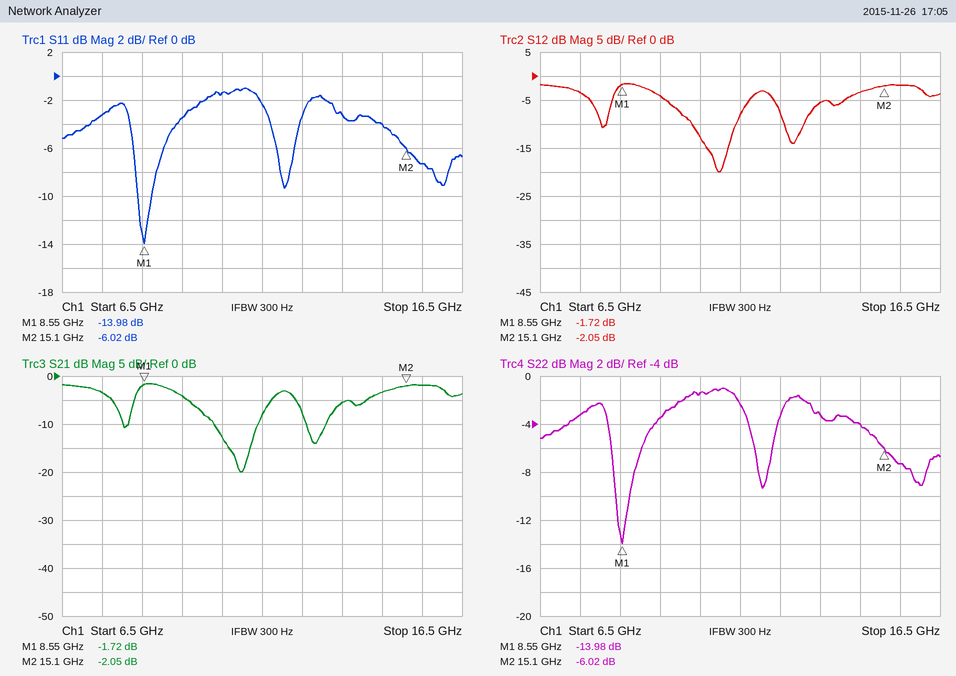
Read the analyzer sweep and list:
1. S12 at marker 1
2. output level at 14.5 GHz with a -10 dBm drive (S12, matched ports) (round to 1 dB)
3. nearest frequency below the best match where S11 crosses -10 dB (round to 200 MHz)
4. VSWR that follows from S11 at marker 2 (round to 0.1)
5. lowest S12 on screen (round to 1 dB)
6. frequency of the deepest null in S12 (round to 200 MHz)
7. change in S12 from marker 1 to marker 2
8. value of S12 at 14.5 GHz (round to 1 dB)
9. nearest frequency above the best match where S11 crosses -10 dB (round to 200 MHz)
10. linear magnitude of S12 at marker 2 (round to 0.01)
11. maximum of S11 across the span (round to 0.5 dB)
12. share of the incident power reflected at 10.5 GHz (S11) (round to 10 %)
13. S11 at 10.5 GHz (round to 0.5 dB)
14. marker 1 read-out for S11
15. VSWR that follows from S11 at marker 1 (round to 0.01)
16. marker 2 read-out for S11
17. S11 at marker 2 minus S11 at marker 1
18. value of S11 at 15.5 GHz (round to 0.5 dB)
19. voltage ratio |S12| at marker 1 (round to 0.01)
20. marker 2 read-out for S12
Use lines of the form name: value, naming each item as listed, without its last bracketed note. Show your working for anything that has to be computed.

S12 at marker 1: -1.72 dB
output level at 14.5 GHz with a -10 dBm drive (S12, matched ports): -10 dBm + (-3 dB) = -13 dBm
nearest frequency below the best match where S11 crosses -10 dB: 8.4 GHz
VSWR that follows from S11 at marker 2: (1 + 0.5000)/(1 − 0.5000) ≈ 3.0
lowest S12 on screen: -20 dB
frequency of the deepest null in S12: 11.0 GHz
change in S12 from marker 1 to marker 2: -2.05 − (-1.72) = -0.33 dB
value of S12 at 14.5 GHz: -3 dB
nearest frequency above the best match where S11 crosses -10 dB: 8.8 GHz
linear magnitude of S12 at marker 2: 10^(-2.05/20) ≈ 0.79
maximum of S11 across the span: -1.0 dB
share of the incident power reflected at 10.5 GHz (S11): 10^(-1.5/10) ≈ 70.8 %, so 70 % to the nearest 10 %
S11 at 10.5 GHz: -1.5 dB
marker 1 read-out for S11: -13.98 dB
VSWR that follows from S11 at marker 1: (1 + 0.2000)/(1 − 0.2000) ≈ 1.50
marker 2 read-out for S11: -6.02 dB
S11 at marker 2 minus S11 at marker 1: -6.02 − (-13.98) = 7.96 dB
value of S11 at 15.5 GHz: -7.5 dB
voltage ratio |S12| at marker 1: 10^(-1.72/20) ≈ 0.82
marker 2 read-out for S12: -2.05 dB
